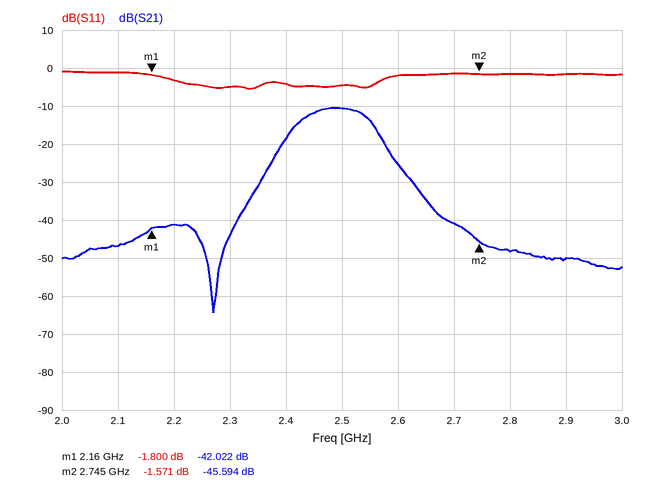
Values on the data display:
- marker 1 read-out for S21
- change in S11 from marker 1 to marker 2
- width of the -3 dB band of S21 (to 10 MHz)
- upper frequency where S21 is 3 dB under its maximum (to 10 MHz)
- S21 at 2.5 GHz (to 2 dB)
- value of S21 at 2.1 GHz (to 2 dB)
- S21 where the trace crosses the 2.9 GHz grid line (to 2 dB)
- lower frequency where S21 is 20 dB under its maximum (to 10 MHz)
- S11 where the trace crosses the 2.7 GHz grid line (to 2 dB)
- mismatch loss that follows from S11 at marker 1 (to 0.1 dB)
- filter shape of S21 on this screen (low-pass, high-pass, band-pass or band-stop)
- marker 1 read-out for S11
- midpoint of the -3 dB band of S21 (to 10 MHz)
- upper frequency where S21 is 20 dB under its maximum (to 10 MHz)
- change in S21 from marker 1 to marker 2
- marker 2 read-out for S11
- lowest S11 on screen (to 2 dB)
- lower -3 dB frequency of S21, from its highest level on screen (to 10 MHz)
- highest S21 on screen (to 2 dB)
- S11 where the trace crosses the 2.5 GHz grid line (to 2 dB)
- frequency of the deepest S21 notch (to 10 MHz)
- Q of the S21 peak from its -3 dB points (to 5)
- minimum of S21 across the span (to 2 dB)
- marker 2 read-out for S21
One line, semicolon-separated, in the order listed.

-42.022 dB; 0.229 dB; 120 MHz; 2.55 GHz; -10 dB; -46 dB; -50 dB; 2.35 GHz; -2 dB; 4.7 dB; band-pass; -1.800 dB; 2.49 GHz; 2.63 GHz; -3.572 dB; -1.571 dB; -6 dB; 2.43 GHz; -10 dB; -4 dB; 2.27 GHz; 20; -64 dB; -45.594 dB
